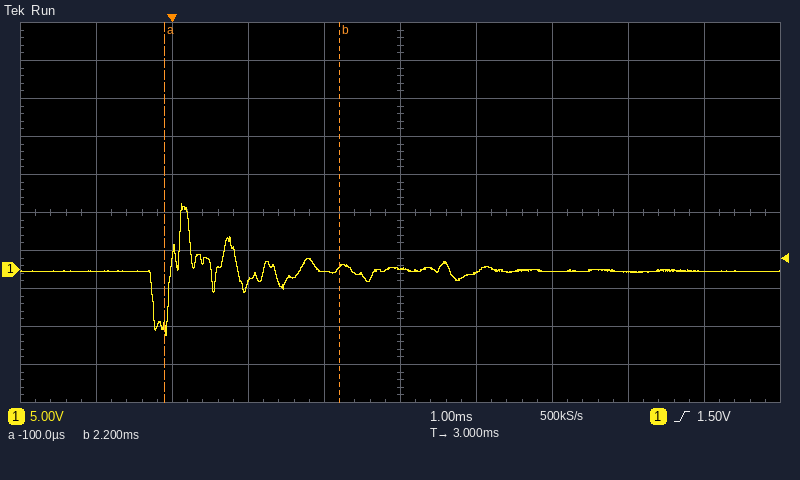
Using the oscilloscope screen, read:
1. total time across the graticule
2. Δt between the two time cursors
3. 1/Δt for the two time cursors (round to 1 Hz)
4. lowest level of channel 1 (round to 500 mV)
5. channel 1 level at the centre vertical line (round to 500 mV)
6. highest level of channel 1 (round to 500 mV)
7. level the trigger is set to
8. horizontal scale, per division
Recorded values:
10 ms
2.3 ms
435 Hz
-8.5 V
0.0 V
8.5 V
1.50 V
1 ms
